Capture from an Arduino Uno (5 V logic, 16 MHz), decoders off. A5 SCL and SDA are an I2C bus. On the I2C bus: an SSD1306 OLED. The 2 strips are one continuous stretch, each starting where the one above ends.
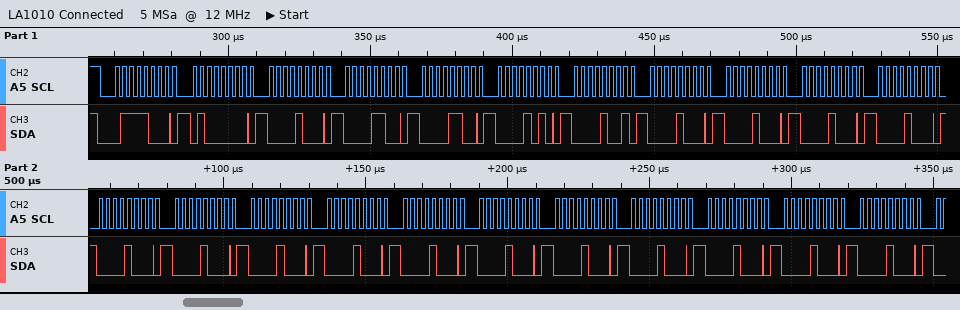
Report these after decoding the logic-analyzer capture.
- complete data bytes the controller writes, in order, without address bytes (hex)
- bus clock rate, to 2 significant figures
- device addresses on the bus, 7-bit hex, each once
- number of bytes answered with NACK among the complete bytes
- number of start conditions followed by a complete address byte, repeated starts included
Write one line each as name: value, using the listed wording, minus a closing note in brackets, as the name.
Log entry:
complete data bytes the controller writes, in order, without address bytes: 40 08 0C 0C 0A 09 08 08 08 08 08 08 08 08 08 08 08 08 08 08 08
bus clock rate, to 2 significant figures: 400 kHz
device addresses on the bus, 7-bit hex, each once: 0x3C
number of bytes answered with NACK among the complete bytes: 0
number of start conditions followed by a complete address byte, repeated starts included: 1
